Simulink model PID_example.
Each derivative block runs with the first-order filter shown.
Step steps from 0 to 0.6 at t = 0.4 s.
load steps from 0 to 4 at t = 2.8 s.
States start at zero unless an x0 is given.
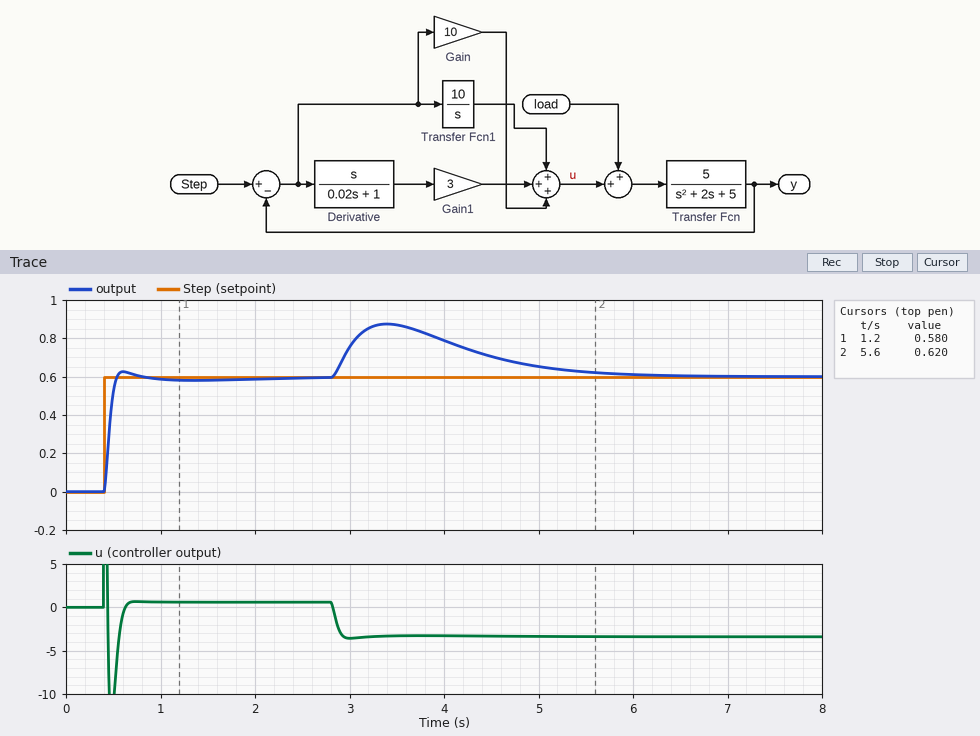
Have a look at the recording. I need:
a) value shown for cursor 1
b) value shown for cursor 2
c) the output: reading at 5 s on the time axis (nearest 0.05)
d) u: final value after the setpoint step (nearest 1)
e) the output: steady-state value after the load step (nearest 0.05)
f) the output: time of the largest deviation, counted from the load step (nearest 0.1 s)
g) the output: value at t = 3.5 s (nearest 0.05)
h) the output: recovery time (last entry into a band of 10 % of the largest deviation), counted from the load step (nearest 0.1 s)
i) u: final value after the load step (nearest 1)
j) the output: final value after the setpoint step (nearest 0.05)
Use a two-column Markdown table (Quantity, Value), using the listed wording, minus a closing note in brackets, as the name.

| Quantity | Value |
|---|---|
| value shown for cursor 1 | 0.580 |
| value shown for cursor 2 | 0.620 |
| the output: reading at 5 s on the time axis | 0.65 |
| u: final value after the setpoint step | 1 |
| the output: steady-state value after the load step | 0.60 |
| the output: time of the largest deviation, counted from the load step | 0.6 s |
| the output: value at t = 3.5 s | 0.85 |
| the output: recovery time (last entry into a band of 10 % of the largest deviation), counted from the load step | 2.6 s |
| u: final value after the load step | -3 |
| the output: final value after the setpoint step | 0.60 |
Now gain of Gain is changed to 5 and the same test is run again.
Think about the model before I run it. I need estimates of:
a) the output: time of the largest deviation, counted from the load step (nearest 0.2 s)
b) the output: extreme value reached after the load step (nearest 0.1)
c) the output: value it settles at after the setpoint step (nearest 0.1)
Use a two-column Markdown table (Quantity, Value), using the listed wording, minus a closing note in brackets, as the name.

| Quantity | Value |
|---|---|
| the output: time of the largest deviation, counted from the load step | 0.8 s |
| the output: extreme value reached after the load step | 1.0 |
| the output: value it settles at after the setpoint step | 0.6 |
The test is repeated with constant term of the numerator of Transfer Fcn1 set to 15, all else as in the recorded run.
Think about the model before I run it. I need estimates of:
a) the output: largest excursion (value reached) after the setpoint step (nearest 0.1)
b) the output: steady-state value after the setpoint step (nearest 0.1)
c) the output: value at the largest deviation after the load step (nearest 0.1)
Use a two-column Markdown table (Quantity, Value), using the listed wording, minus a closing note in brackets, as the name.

| Quantity | Value |
|---|---|
| the output: largest excursion (value reached) after the setpoint step | 0.6 |
| the output: steady-state value after the setpoint step | 0.6 |
| the output: value at the largest deviation after the load step | 0.9 |
